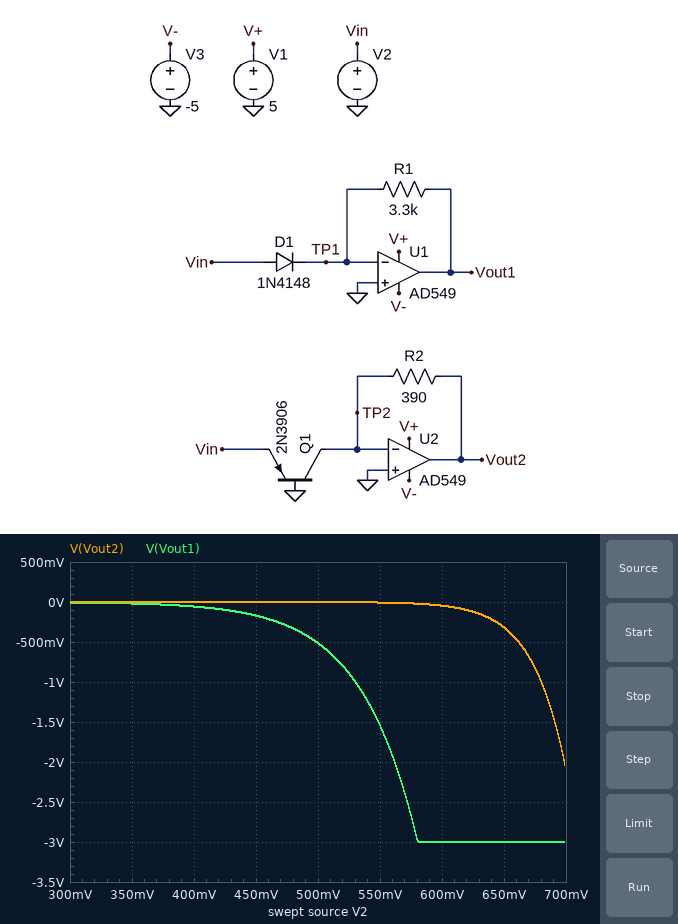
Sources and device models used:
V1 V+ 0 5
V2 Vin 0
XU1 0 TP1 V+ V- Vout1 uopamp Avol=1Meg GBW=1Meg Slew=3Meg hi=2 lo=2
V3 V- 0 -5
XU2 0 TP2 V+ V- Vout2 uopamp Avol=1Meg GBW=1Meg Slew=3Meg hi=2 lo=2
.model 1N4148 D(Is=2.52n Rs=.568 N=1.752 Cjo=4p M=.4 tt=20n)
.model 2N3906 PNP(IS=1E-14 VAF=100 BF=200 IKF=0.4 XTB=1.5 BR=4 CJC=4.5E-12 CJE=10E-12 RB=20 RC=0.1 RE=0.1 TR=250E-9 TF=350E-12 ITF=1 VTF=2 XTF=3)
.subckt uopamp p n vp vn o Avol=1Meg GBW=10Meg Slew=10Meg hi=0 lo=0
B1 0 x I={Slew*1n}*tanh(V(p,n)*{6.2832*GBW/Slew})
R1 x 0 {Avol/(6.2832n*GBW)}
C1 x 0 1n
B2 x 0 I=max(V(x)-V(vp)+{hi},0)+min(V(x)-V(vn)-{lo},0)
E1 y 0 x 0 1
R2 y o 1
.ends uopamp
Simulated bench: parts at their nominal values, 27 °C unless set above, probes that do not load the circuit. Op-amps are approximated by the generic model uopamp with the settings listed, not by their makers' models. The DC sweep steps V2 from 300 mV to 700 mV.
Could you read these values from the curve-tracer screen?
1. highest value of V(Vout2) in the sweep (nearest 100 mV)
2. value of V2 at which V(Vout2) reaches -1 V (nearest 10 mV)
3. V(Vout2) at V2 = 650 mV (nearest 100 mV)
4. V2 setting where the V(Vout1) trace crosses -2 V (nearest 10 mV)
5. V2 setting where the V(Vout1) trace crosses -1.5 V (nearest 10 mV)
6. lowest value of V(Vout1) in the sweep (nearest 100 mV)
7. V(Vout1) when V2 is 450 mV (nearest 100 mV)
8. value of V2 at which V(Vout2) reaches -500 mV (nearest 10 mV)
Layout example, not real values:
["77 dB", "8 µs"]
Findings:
["0 V", "680 mV", "-300 mV", "560 mV", "550 mV", "-3.0 V", "-200 mV", "660 mV"]
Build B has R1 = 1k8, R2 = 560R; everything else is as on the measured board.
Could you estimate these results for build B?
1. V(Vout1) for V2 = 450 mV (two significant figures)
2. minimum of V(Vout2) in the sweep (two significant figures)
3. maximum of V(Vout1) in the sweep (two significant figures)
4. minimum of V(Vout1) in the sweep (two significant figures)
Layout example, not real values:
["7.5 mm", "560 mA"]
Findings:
["-93 mV", "-3.0 V", "-3.4 mV", "-3.0 V"]
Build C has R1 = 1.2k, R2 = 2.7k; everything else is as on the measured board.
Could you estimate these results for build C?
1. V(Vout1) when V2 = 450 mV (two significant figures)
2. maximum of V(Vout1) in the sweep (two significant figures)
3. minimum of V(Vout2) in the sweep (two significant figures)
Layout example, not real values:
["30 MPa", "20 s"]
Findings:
["-62 mV", "-2.3 mV", "-3.0 V"]
